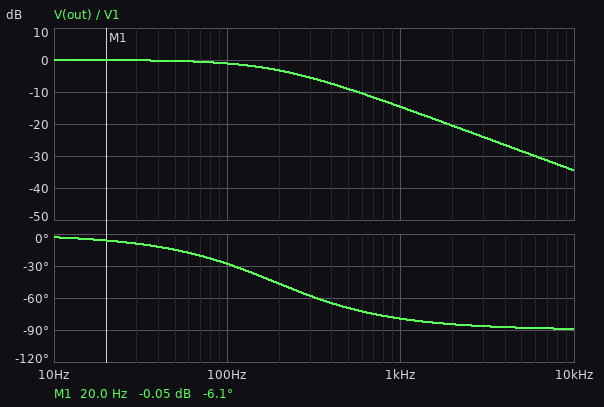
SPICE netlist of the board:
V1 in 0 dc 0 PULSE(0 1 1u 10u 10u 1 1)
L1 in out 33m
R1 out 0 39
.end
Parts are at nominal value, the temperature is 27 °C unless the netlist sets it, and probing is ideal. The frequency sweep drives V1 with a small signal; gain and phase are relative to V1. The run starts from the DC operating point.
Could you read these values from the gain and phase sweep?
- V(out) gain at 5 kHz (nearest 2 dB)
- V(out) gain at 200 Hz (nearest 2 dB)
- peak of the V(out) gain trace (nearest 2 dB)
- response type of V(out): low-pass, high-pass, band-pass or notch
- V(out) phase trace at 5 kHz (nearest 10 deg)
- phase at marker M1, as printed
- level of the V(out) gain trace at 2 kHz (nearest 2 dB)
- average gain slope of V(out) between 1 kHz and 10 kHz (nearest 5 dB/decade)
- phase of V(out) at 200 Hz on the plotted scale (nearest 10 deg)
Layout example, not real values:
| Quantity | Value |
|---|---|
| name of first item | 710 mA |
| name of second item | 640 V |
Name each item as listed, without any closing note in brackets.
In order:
| Quantity | Value |
|---|---|
| V(out) gain at 5 kHz | -28 dB |
| V(out) gain at 200 Hz | -4 dB |
| peak of the V(out) gain trace | 0 dB |
| response type of V(out): low-pass, high-pass, band-pass or notch | low-pass |
| V(out) phase trace at 5 kHz | -90 deg |
| phase at marker M1, as printed | -6.1 deg |
| level of the V(out) gain trace at 2 kHz | -20 dB |
| average gain slope of V(out) between 1 kHz and 10 kHz | -20 dB/decade |
| phase of V(out) at 200 Hz on the plotted scale | -50 deg |
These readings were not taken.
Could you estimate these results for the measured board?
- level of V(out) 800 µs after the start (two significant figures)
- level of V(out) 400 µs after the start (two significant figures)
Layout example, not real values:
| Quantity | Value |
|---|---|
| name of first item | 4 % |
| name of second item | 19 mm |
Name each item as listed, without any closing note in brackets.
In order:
| Quantity | Value |
|---|---|
| level of V(out) 800 µs after the start | 610 mV |
| level of V(out) 400 µs after the start | 370 mV |
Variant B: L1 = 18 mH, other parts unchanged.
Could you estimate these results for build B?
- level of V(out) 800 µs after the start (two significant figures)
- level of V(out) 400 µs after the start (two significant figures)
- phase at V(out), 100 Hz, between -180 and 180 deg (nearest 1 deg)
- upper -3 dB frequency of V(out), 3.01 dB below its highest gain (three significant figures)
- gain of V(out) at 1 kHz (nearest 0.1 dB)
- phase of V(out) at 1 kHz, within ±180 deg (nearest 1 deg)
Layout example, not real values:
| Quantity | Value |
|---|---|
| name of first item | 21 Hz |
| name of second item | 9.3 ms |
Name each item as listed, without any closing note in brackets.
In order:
| Quantity | Value |
|---|---|
| level of V(out) 800 µs after the start | 820 mV |
| level of V(out) 400 µs after the start | 570 mV |
| phase at V(out), 100 Hz, between -180 and 180 deg | -16 deg |
| upper -3 dB frequency of V(out), 3.01 dB below its highest gain | 345 Hz |
| gain of V(out) at 1 kHz | -9.7 dB |
| phase of V(out) at 1 kHz, within ±180 deg | -71 deg |
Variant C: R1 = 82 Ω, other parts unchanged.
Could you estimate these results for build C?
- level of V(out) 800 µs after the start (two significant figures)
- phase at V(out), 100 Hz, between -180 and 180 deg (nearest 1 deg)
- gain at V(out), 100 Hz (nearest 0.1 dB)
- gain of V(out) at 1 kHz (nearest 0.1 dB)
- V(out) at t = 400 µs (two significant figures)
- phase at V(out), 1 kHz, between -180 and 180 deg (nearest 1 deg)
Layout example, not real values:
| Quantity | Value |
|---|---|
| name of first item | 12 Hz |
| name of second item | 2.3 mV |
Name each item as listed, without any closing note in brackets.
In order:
| Quantity | Value |
|---|---|
| level of V(out) 800 µs after the start | 860 mV |
| phase at V(out), 100 Hz, between -180 and 180 deg | -14 deg |
| gain at V(out), 100 Hz | -0.3 dB |
| gain of V(out) at 1 kHz | -8.7 dB |
| V(out) at t = 400 µs | 620 mV |
| phase at V(out), 1 kHz, between -180 and 180 deg | -68 deg |
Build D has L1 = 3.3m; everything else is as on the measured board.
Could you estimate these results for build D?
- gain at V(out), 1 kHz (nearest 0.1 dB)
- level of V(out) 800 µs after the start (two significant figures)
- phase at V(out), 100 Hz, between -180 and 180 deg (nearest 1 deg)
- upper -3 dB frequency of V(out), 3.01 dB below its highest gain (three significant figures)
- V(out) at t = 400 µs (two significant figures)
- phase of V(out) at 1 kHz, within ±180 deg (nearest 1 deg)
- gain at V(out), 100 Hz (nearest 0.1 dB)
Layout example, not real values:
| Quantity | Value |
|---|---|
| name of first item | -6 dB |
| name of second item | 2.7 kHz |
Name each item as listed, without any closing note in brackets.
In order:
| Quantity | Value |
|---|---|
| gain at V(out), 1 kHz | -1.1 dB |
| level of V(out) 800 µs after the start | 1.0 V |
| phase at V(out), 100 Hz, between -180 and 180 deg | -3 deg |
| upper -3 dB frequency of V(out), 3.01 dB below its highest gain | 1.88 kHz |
| V(out) at t = 400 µs | 990 mV |
| phase of V(out) at 1 kHz, within ±180 deg | -28 deg |
| gain at V(out), 100 Hz | 0 dB |
